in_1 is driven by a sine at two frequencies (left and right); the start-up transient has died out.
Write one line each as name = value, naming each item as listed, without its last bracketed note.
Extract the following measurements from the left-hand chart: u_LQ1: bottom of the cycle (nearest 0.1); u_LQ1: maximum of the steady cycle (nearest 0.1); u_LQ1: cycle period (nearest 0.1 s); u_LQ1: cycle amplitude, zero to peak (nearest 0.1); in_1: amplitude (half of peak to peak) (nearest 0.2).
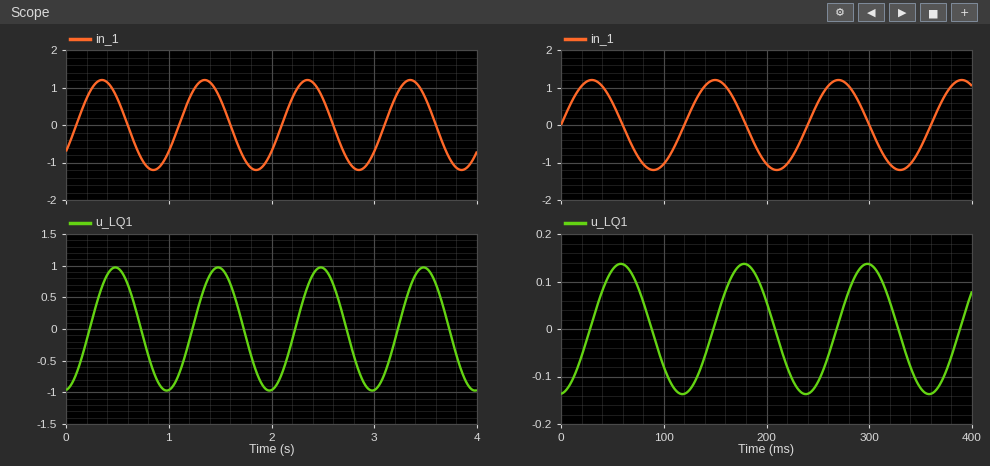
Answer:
u_LQ1: bottom of the cycle = -1.0
u_LQ1: maximum of the steady cycle = 1.0
u_LQ1: cycle period = 1.0 s
u_LQ1: cycle amplitude, zero to peak = 1.0
in_1: amplitude (half of peak to peak) = 1.2
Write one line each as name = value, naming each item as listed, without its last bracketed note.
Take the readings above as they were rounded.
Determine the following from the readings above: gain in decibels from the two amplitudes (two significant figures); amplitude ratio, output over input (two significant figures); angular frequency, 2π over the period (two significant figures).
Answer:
gain in decibels from the two amplitudes = -1.6 dB
amplitude ratio, output over input = 0.83
angular frequency, 2π over the period = 6.3 rad/s
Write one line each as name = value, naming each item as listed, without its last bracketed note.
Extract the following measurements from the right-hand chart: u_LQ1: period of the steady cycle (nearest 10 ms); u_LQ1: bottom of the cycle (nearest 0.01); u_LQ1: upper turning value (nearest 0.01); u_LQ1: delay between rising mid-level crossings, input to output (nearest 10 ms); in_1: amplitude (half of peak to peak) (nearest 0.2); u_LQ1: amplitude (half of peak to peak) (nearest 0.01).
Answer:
u_LQ1: period of the steady cycle = 120 ms
u_LQ1: bottom of the cycle = -0.14
u_LQ1: upper turning value = 0.14
u_LQ1: delay between rising mid-level crossings, input to output = 30 ms
in_1: amplitude (half of peak to peak) = 1.2
u_LQ1: amplitude (half of peak to peak) = 0.14
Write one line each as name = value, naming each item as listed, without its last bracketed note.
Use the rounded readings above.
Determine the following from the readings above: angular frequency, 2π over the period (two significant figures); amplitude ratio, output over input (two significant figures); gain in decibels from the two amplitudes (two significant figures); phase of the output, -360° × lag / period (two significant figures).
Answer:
angular frequency, 2π over the period = 0.052 rad/ms
amplitude ratio, output over input = 0.12
gain in decibels from the two amplitudes = -19 dB
phase of the output, -360° × lag / period = -90°
